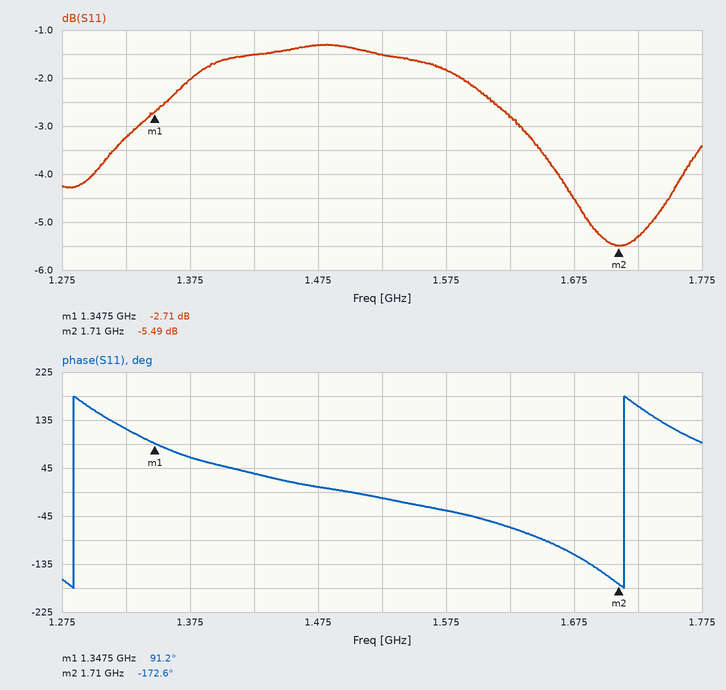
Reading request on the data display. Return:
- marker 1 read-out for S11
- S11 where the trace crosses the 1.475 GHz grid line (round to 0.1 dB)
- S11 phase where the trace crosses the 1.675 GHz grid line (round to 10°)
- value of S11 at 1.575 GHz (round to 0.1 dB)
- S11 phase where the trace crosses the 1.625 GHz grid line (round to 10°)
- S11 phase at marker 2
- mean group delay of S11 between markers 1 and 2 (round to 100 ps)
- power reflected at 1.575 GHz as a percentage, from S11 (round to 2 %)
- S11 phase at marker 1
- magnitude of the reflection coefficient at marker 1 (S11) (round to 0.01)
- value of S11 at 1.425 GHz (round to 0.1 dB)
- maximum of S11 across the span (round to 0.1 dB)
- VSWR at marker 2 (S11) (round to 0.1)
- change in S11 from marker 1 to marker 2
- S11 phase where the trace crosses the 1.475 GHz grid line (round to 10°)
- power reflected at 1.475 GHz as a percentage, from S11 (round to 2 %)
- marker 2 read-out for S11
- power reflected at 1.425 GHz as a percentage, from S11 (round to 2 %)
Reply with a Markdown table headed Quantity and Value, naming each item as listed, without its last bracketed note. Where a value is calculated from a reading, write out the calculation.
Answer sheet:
| Quantity | Value |
|---|---|
| marker 1 read-out for S11 | -2.71 dB |
| S11 where the trace crosses the 1.475 GHz grid line | -1.3 dB |
| S11 phase where the trace crosses the 1.675 GHz grid line | -120° |
| value of S11 at 1.575 GHz | -1.8 dB |
| S11 phase where the trace crosses the 1.625 GHz grid line | -70° |
| S11 phase at marker 2 | -172.6° |
| mean group delay of S11 between markers 1 and 2 | −(-172.6° − (91.2°))/(360° × 362.5 MHz) ≈ 2.0 ns |
| power reflected at 1.575 GHz as a percentage, from S11 | 10^(-1.8/10) ≈ 66 % |
| S11 phase at marker 1 | 91.2° |
| magnitude of the reflection coefficient at marker 1 (S11) | 10^(-2.71/20) ≈ 0.73 |
| value of S11 at 1.425 GHz | -1.5 dB |
| maximum of S11 across the span | -1.3 dB |
| VSWR at marker 2 (S11) | (1 + 0.5315)/(1 − 0.5315) ≈ 3.3 |
| change in S11 from marker 1 to marker 2 | -5.49 − (-2.71) = -2.78 dB |
| S11 phase where the trace crosses the 1.475 GHz grid line | 10° |
| power reflected at 1.475 GHz as a percentage, from S11 | 10^(-1.3/10) ≈ 74 % |
| marker 2 read-out for S11 | -5.49 dB |
| power reflected at 1.425 GHz as a percentage, from S11 | 10^(-1.5/10) ≈ 70.8 %, so 70 % to the nearest 2 % |
